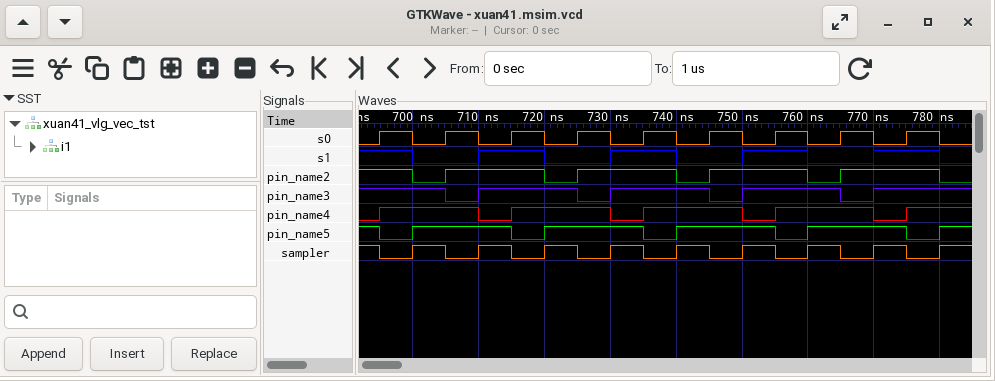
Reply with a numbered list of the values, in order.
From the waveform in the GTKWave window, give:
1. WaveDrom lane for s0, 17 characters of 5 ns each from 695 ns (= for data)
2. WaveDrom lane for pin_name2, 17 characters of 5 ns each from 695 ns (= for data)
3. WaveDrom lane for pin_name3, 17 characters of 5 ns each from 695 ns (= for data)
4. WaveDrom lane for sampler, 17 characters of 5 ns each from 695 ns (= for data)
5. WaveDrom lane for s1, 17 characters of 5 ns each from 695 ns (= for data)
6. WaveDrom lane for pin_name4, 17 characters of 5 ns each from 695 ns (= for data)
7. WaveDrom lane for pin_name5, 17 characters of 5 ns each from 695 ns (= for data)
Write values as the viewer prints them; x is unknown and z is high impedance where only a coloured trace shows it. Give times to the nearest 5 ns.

1. {name: 's0', wave: '10101010101010101'}
2. {name: 'pin_name2', wave: '101..01..01..01..'}
3. {name: 'pin_name3', wave: '1.01..01..01..01.'}
4. {name: 'sampler', wave: '01010101010101010'}
5. {name: 's1', wave: '10.1.0.1.0.1.0.1.'}
6. {name: 'pin_name4', wave: '1..01..01..01..01'}
7. {name: 'pin_name5', wave: '01..01..01..01..0'}
